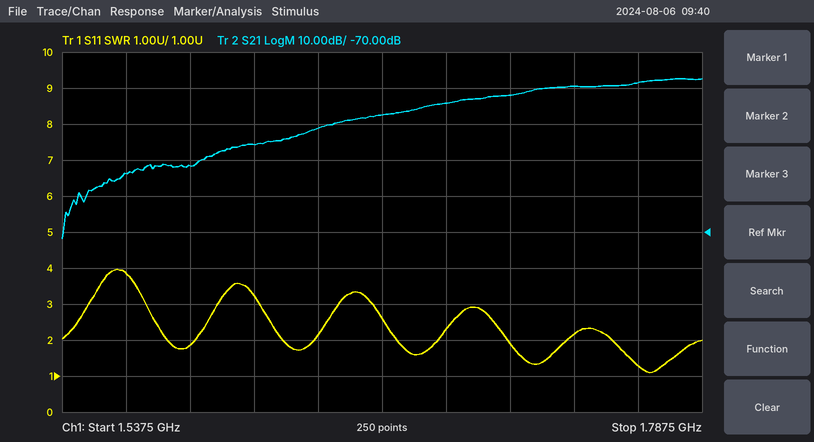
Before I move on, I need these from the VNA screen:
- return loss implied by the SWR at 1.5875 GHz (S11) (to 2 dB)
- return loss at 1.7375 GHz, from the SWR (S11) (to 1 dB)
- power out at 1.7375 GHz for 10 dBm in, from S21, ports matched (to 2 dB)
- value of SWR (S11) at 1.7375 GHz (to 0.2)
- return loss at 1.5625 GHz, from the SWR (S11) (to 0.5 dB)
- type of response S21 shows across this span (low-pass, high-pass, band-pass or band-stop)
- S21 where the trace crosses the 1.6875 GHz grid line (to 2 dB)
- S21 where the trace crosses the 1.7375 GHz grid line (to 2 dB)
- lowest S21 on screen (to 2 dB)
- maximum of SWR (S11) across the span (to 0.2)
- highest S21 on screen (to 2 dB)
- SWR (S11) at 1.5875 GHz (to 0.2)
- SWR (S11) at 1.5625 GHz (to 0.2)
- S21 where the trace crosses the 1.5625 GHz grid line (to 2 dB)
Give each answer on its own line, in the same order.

10 dB
9 dB
-20 dBm
2.2
4.5 dB
high-pass
-34 dB
-30 dB
-72 dB
4.0
-28 dB
1.8
3.8
-54 dB
